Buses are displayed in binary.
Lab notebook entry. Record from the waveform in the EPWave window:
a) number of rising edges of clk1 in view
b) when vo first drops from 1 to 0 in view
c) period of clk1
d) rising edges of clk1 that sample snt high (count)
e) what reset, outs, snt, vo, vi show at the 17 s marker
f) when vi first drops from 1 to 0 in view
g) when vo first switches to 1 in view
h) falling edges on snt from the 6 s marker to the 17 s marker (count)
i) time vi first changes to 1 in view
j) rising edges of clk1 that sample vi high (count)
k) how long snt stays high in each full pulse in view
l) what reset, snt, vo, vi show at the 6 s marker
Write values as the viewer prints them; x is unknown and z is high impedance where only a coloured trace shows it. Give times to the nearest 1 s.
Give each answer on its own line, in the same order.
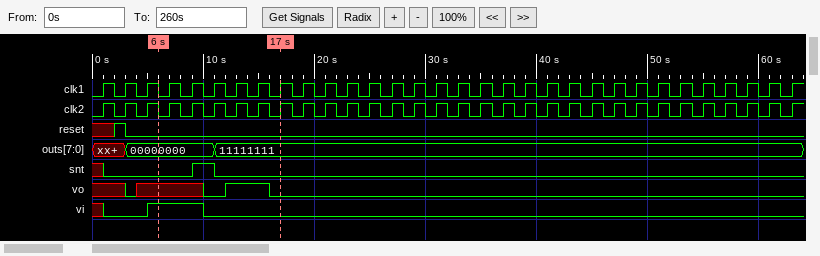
32
16 s
2 s
1
reset=0, outs=11111111, snt=0, vo=0, vi=0
10 s
12 s
1
5 s
2
2 s
reset=0, snt=0, vo=x, vi=1
